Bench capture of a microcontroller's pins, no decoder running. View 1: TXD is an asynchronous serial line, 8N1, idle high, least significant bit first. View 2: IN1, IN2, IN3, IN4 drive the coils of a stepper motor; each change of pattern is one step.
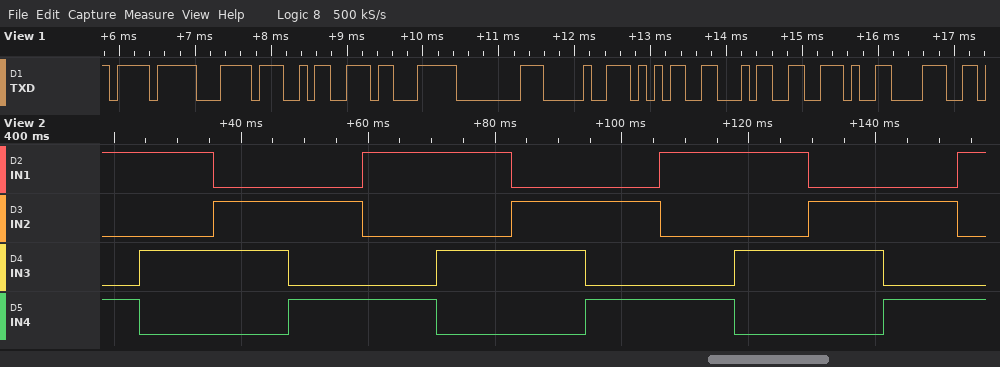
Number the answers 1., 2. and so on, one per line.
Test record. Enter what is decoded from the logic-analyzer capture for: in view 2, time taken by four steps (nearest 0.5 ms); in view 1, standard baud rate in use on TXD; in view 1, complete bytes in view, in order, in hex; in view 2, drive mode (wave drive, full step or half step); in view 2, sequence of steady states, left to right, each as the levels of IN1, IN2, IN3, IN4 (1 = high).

1. 47.0 ms
2. 9600 baud
3. EF BC 9A E3 80 90 35 34 2E 38
4. full step
5. 1001 1010 0110 0101 1001 1010 0110 0101 1001 1010 0110 0101 1001
